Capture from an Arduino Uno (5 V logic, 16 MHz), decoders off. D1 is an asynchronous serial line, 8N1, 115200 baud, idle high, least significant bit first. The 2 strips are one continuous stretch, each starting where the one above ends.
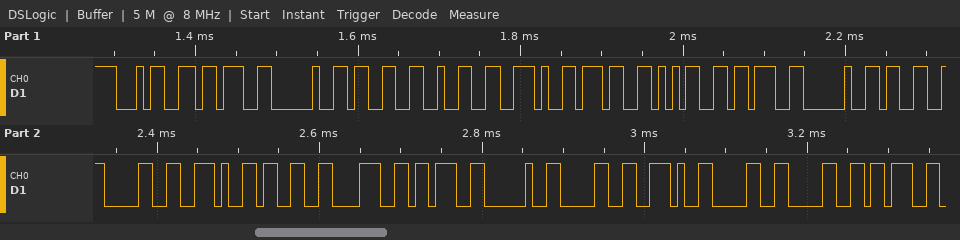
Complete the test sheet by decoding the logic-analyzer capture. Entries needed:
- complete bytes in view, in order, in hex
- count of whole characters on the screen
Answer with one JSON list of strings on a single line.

["0x34 0x3B 0x20 0x33 0x32 0x2E 0x37 0x35 0x3B 0x20 0x33 0x30 0x2E 0x33 0x38 0x3B 0x20 0x30 0x2E 0x30 0x30 0x3B", "22"]
